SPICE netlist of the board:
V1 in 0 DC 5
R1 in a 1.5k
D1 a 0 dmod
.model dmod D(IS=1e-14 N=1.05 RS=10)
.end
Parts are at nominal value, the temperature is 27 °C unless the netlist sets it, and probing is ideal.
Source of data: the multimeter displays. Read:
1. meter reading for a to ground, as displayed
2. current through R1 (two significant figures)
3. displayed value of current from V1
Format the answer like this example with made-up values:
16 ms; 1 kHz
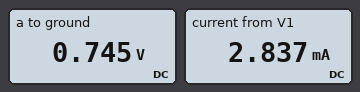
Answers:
0.745 V; 2.8 mA; 2.837 mA
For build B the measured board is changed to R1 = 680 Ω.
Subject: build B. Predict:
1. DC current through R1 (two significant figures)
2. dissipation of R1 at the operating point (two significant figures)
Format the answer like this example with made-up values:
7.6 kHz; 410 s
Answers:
6.2 mA; 26 mW
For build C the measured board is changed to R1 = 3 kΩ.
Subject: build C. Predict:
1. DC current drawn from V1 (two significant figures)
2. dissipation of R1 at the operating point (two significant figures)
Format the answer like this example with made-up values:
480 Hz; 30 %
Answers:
1.4 mA; 6.1 mW
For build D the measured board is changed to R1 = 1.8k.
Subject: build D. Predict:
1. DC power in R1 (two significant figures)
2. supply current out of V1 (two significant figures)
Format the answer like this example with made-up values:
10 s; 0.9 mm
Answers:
10 mW; 2.4 mA
